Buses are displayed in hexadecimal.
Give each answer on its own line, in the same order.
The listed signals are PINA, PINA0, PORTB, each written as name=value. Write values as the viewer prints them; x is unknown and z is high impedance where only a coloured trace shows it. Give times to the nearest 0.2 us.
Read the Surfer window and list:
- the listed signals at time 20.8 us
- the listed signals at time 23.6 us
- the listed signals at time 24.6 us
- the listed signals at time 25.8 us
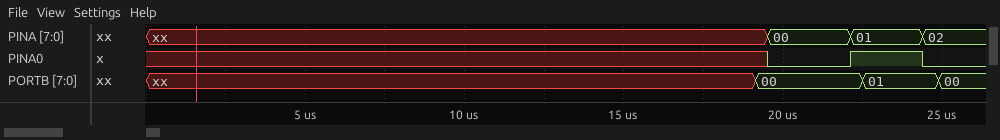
PINA=00, PINA0=0, PORTB=00
PINA=01, PINA0=1, PORTB=01
PINA=02, PINA0=0, PORTB=01
PINA=02, PINA0=0, PORTB=00
